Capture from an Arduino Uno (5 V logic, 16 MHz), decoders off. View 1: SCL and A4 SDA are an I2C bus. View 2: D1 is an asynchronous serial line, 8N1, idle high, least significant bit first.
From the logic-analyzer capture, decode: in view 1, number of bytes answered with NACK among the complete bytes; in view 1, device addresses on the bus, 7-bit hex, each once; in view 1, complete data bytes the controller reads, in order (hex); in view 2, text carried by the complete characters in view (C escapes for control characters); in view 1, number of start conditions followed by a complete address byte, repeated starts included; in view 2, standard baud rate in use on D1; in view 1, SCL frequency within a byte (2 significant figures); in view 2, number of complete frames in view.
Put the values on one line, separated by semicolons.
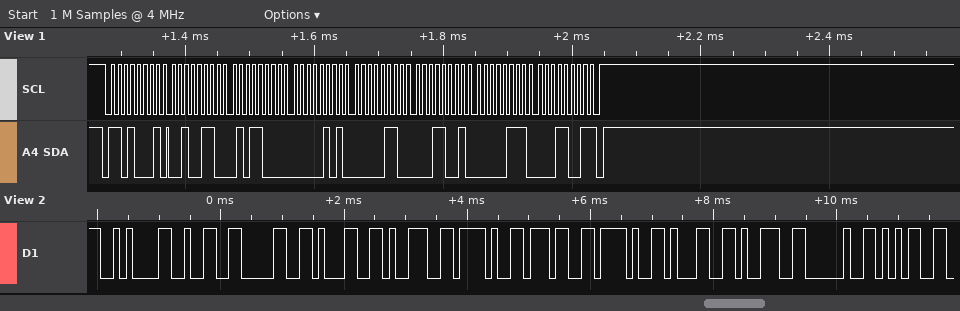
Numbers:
1; 0x68; 26 58 05 06 19 07 19; "\n2019/7/19 5"; 1; 9600 baud; 100 kHz; 12
